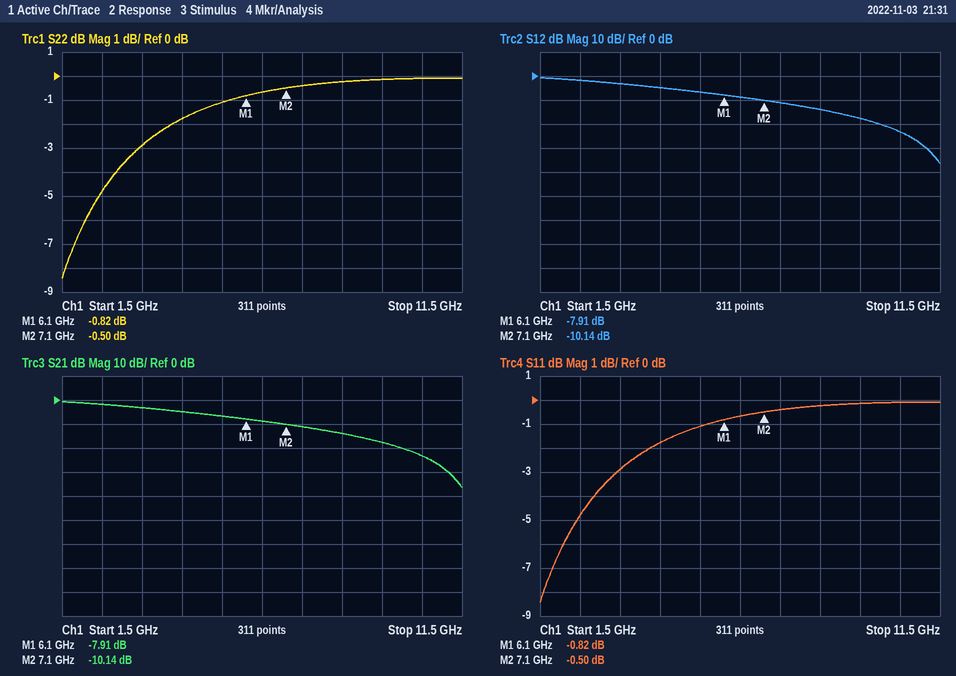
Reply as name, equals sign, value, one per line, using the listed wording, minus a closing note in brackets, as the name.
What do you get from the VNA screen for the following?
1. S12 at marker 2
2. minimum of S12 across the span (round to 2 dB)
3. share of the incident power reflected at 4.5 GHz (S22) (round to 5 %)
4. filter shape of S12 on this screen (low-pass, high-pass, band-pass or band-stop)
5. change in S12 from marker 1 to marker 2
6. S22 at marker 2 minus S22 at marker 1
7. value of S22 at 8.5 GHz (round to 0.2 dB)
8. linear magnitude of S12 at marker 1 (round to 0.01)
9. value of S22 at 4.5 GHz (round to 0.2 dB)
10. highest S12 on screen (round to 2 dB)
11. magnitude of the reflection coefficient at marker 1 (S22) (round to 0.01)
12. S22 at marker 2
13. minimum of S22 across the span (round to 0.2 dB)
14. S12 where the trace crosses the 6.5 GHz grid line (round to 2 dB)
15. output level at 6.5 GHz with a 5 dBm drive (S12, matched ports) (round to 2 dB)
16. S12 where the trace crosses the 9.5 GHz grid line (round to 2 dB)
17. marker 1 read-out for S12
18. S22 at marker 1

S12 at marker 2 = -10.14 dB
minimum of S12 across the span = -36 dB
share of the incident power reflected at 4.5 GHz (S22) = 65 %
filter shape of S12 on this screen = low-pass
change in S12 from marker 1 to marker 2 = -2.23 dB
S22 at marker 2 minus S22 at marker 1 = 0.32 dB
value of S22 at 8.5 GHz = -0.2 dB
linear magnitude of S12 at marker 1 = 0.40
value of S22 at 4.5 GHz = -1.8 dB
highest S12 on screen = 0 dB
magnitude of the reflection coefficient at marker 1 (S22) = 0.91
S22 at marker 2 = -0.50 dB
minimum of S22 across the span = -8.4 dB
S12 where the trace crosses the 6.5 GHz grid line = -8 dB
output level at 6.5 GHz with a 5 dBm drive (S12, matched ports) = -4 dBm
S12 where the trace crosses the 9.5 GHz grid line = -18 dB
marker 1 read-out for S12 = -7.91 dB
S22 at marker 1 = -0.82 dB
